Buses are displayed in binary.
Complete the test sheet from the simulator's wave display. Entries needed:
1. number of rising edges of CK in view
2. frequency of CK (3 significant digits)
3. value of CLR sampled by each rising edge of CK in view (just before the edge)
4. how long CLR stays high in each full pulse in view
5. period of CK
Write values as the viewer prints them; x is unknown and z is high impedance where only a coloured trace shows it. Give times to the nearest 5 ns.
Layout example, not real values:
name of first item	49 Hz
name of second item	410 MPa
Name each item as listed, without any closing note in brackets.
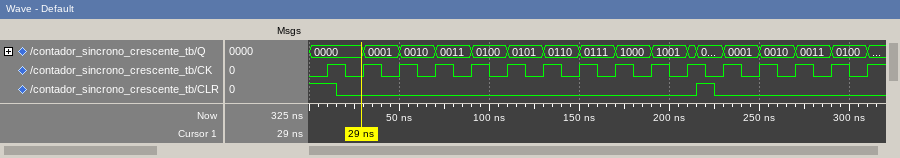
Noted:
number of rising edges of CK in view	16
frequency of CK	50.0 MHz
value of CLR sampled by each rising edge of CK in view	1 0 0 0 0 0 0 0 0 0 0 0 0 0 0 0
how long CLR stays high in each full pulse in view	10 ns
period of CK	20 ns
